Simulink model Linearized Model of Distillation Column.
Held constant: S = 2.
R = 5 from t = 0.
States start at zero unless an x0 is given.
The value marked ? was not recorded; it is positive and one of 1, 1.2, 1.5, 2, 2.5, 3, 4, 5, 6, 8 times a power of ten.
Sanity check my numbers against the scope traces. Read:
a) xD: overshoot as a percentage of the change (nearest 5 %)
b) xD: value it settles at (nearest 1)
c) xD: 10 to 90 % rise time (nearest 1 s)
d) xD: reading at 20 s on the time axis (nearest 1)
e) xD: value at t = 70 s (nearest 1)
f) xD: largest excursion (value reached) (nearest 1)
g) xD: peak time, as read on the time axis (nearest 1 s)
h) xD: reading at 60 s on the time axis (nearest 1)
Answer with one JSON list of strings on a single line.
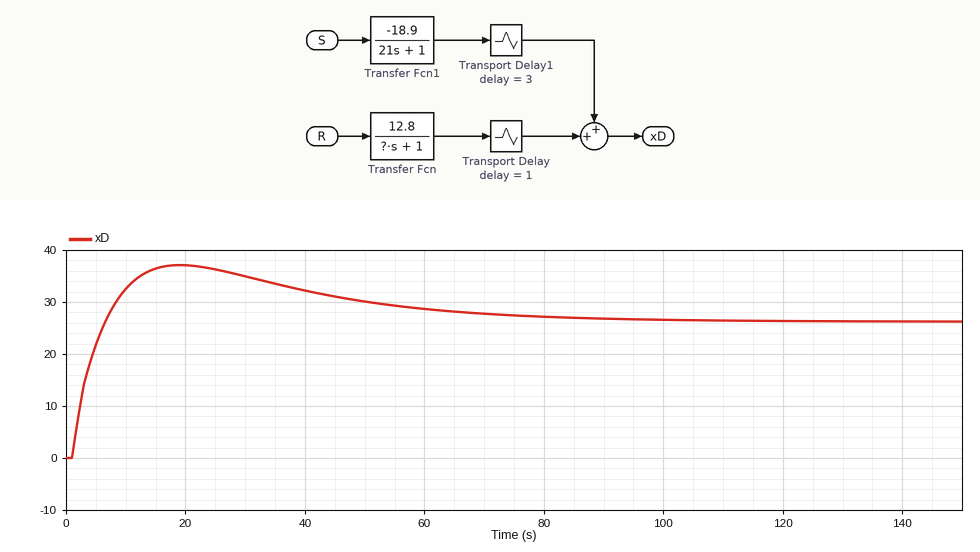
["40 %", "26", "4 s", "37", "28", "37", "19 s", "29"]
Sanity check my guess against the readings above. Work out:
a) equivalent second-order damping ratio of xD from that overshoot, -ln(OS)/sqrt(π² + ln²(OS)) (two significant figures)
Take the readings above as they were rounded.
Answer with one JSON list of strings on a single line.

["0.28"]
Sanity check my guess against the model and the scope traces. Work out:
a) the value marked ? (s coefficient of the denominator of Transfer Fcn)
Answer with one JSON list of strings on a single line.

["8"]
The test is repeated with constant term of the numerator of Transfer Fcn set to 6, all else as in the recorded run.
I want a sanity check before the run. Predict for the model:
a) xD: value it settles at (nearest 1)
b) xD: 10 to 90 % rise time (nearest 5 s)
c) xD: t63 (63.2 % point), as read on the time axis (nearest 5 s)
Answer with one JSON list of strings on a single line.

["-8", "45 s", "55 s"]
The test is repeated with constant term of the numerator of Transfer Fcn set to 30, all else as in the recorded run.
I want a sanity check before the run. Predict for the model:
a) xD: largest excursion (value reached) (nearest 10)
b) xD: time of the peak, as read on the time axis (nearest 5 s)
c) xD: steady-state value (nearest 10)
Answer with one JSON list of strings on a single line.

["120", "30 s", "110"]
